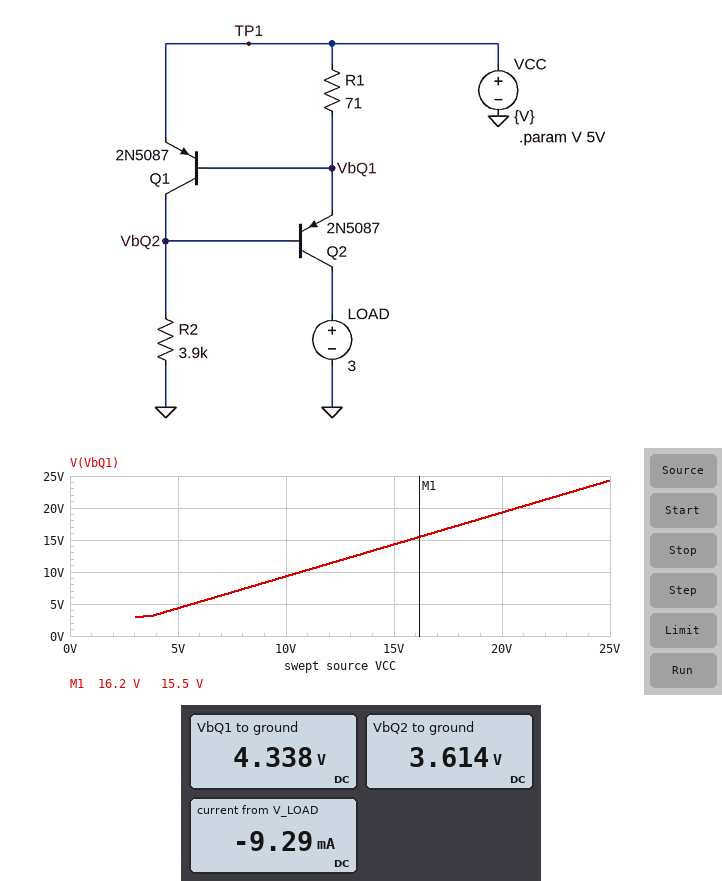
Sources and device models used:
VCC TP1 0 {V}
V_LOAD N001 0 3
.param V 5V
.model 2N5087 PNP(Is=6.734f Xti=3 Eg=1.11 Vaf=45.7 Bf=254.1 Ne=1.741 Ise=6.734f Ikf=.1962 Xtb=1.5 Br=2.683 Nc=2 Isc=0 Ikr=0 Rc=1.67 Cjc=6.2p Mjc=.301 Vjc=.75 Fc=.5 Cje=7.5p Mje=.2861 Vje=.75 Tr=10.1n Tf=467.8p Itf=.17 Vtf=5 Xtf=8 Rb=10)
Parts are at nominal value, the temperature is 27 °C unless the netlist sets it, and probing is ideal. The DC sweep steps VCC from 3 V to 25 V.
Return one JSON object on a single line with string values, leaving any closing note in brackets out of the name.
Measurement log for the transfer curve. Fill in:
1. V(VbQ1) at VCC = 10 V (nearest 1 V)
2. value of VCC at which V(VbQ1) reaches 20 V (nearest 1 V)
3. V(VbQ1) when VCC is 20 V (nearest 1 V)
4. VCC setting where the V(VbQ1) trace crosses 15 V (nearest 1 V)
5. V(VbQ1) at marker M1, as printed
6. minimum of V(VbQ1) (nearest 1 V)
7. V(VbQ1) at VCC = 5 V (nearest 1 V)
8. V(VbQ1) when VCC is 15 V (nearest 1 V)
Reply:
{"V(VbQ1) at VCC = 10 V": "9 V", "value of VCC at which V(VbQ1) reaches 20 V": "21 V", "V(VbQ1) when VCC is 20 V": "19 V", "VCC setting where the V(VbQ1) trace crosses 15 V": "16 V", "V(VbQ1) at marker M1, as printed": "15.5 V", "minimum of V(VbQ1)": "3 V", "V(VbQ1) at VCC = 5 V": "4 V", "V(VbQ1) when VCC is 15 V": "14 V"}
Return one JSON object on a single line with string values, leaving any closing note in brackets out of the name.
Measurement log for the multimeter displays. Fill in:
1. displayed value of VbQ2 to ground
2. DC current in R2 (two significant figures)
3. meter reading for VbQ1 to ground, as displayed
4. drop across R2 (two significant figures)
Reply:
{"displayed value of VbQ2 to ground": "3.614 V", "DC current in R2": "930 µA", "meter reading for VbQ1 to ground, as displayed": "4.338 V", "drop across R2": "3.6 V"}
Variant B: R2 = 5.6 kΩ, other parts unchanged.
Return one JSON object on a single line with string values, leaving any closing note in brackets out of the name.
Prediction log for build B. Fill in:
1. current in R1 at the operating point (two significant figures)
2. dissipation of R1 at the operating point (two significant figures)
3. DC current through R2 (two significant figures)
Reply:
{"current in R1 at the operating point": "9.2 mA", "dissipation of R1 at the operating point": "6.0 mW", "DC current through R2": "650 µA"}
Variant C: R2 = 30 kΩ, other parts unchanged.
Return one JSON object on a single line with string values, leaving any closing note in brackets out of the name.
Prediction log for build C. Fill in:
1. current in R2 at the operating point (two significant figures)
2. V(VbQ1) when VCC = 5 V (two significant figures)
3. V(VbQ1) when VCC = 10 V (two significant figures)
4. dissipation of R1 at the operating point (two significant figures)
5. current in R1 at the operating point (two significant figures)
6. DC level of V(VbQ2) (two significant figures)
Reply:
{"current in R2 at the operating point": "120 µA", "V(VbQ1) when VCC = 5 V": "4.4 V", "V(VbQ1) when VCC = 10 V": "9.4 V", "dissipation of R1 at the operating point": "5.1 mW", "current in R1 at the operating point": "8.5 mA", "DC level of V(VbQ2)": "3.7 V"}
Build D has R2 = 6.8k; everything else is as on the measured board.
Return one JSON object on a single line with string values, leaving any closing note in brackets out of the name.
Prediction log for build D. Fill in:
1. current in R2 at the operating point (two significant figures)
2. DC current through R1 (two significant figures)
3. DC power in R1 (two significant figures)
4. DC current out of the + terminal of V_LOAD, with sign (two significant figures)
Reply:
{"current in R2 at the operating point": "530 µA", "DC current through R1": "9.1 mA", "DC power in R1": "5.9 mW", "DC current out of the + terminal of V_LOAD, with sign": "-9.1 mA"}
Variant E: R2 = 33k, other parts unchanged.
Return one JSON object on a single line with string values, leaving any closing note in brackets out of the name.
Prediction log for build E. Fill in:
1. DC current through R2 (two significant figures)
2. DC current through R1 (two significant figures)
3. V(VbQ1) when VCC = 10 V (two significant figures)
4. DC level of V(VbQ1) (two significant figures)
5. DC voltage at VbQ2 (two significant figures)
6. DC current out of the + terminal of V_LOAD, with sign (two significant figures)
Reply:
{"DC current through R2": "110 µA", "DC current through R1": "8.4 mA", "V(VbQ1) when VCC = 10 V": "9.4 V", "DC level of V(VbQ1)": "4.4 V", "DC voltage at VbQ2": "3.7 V", "DC current out of the + terminal of V_LOAD, with sign": "-8.4 mA"}
